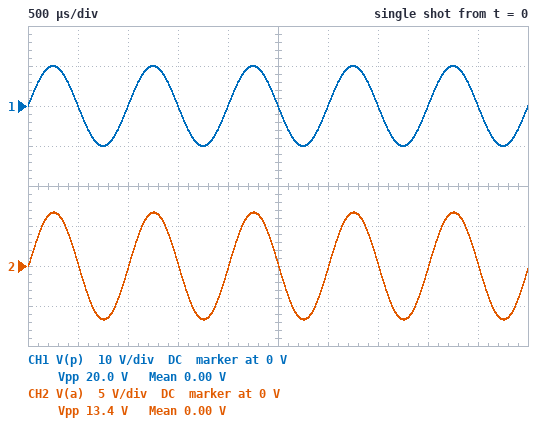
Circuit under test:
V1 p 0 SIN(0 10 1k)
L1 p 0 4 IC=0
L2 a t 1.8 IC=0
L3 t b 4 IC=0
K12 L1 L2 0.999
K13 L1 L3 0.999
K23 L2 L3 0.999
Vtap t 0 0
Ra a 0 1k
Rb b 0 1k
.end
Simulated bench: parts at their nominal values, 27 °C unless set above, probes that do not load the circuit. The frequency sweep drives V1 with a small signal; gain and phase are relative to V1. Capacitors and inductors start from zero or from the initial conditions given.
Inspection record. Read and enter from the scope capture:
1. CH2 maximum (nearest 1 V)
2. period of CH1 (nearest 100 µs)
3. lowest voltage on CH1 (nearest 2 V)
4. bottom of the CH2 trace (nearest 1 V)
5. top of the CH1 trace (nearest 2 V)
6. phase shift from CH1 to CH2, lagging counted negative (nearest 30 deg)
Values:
7 V
1.0 ms
-10 V
-7 V
10 V
0 deg
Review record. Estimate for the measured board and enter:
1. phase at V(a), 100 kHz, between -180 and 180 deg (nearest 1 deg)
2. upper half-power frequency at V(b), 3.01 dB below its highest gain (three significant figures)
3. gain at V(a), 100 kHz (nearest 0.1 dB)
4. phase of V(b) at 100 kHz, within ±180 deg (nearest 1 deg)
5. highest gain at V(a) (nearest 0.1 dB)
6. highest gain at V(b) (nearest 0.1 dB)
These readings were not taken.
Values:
-68 deg
16.8 kHz
-15.2 dB
93 deg
-3.5 dB
0 dB
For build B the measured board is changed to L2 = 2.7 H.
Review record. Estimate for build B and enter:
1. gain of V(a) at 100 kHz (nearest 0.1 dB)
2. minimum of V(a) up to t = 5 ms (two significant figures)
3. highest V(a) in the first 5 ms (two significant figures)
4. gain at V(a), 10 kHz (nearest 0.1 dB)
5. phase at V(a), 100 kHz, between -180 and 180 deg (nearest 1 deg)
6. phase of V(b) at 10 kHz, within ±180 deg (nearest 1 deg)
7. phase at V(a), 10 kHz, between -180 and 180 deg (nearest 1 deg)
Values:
-16.3 dB
-8.2 V
8.2 V
-3.1 dB
-76 deg
146 deg
-30 deg
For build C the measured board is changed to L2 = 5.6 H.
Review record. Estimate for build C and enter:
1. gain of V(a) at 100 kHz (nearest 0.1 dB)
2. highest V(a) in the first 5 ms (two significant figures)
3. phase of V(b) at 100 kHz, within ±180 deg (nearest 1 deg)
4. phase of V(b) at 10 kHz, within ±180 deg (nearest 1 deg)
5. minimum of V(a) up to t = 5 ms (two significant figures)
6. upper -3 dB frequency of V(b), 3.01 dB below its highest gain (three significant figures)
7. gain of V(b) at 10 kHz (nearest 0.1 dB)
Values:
-18.9 dB
12 V
99 deg
141 deg
-12 V
11.4 kHz
-2.5 dB
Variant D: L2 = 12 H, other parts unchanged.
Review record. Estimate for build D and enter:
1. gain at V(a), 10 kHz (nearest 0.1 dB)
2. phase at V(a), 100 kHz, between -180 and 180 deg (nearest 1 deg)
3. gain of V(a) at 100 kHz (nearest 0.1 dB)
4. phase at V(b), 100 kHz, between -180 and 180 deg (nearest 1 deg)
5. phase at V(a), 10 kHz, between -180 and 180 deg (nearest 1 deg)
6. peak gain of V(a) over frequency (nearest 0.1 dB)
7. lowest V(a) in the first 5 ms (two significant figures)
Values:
-1.2 dB
-92 deg
-22.1 dB
102 deg
-64 deg
4.8 dB
-17 V
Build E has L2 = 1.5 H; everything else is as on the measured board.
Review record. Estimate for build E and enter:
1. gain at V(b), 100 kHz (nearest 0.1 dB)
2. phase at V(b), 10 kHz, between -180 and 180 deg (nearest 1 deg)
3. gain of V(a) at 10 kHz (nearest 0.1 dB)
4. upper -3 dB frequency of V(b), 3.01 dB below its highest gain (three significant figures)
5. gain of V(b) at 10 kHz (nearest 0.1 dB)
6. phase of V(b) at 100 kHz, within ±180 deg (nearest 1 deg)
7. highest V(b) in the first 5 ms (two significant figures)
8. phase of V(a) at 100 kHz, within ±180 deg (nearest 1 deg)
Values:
-16.5 dB
149 deg
-5.3 dB
17.3 kHz
-1.2 dB
92 deg
10 V
-63 deg
